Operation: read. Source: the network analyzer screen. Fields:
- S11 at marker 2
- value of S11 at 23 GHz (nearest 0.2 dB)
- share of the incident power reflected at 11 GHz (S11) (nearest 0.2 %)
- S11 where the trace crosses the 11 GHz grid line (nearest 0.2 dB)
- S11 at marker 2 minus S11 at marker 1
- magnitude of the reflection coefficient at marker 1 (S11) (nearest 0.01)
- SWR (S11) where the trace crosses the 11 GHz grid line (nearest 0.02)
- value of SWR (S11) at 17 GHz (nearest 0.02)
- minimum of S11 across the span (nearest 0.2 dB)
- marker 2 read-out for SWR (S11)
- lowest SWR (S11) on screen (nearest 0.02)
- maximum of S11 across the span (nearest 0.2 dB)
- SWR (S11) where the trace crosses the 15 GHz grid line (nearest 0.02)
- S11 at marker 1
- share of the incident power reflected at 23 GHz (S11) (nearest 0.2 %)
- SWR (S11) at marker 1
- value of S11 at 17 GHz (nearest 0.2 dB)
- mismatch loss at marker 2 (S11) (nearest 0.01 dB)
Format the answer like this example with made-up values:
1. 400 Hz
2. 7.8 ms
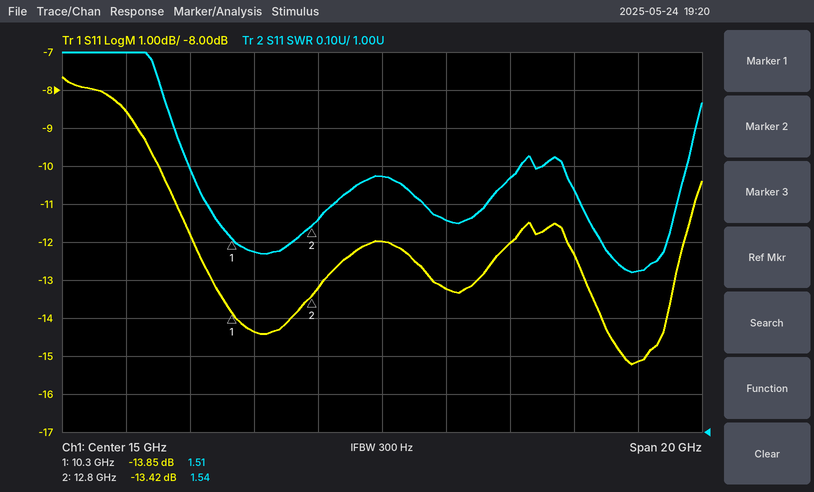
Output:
1. -13.42 dB
2. -15.2 dB
3. 3.6 %
4. -14.4 dB
5. 0.43 dB
6. 0.20
7. 1.48
8. 1.56
9. -15.2 dB
10. 1.54
11. 1.42
12. -7.6 dB
13. 1.68
14. -13.85 dB
15. 3.0 %
16. 1.51
17. -13.2 dB
18. 0.20 dB
